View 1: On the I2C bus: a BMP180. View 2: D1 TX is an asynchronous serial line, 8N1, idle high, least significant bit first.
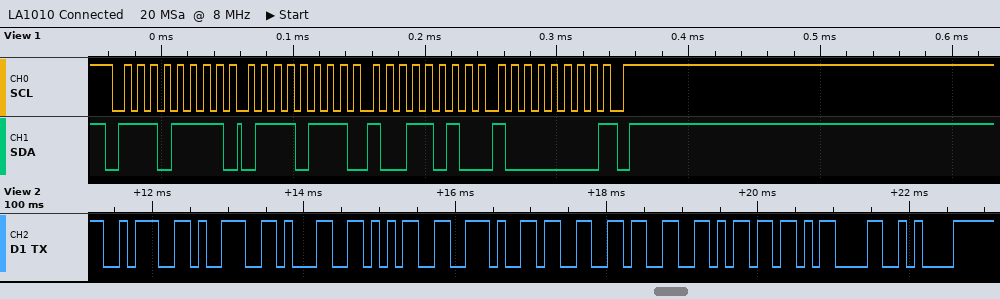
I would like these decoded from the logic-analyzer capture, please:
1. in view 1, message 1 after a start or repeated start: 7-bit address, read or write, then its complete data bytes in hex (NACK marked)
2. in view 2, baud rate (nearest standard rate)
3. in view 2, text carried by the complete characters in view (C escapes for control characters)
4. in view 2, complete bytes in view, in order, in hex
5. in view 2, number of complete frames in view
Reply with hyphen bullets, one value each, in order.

- 0x77 read: 77 9A 80 NACK
- 9600 baud
- ":915.33m\r\n"
- 3A 39 31 35 2E 33 33 6D 0D 0A
- 10
